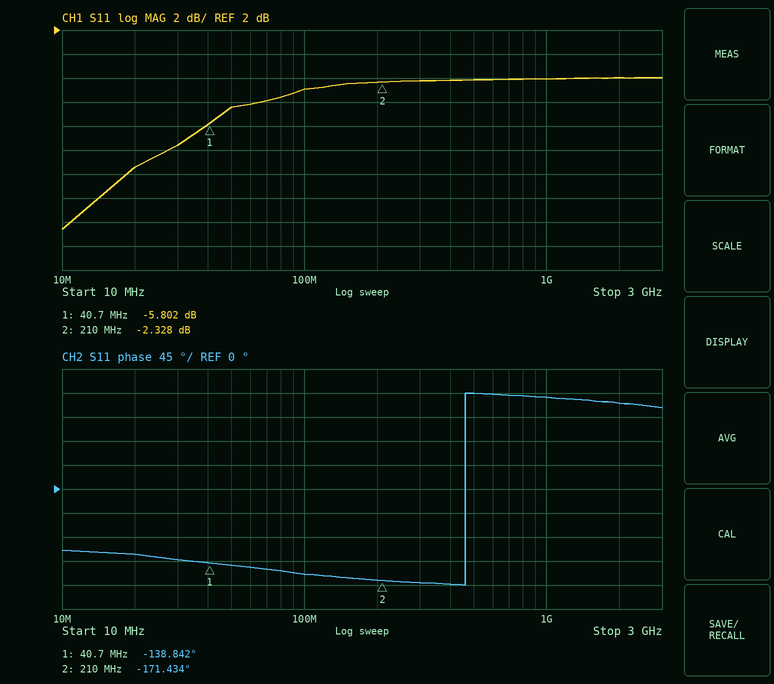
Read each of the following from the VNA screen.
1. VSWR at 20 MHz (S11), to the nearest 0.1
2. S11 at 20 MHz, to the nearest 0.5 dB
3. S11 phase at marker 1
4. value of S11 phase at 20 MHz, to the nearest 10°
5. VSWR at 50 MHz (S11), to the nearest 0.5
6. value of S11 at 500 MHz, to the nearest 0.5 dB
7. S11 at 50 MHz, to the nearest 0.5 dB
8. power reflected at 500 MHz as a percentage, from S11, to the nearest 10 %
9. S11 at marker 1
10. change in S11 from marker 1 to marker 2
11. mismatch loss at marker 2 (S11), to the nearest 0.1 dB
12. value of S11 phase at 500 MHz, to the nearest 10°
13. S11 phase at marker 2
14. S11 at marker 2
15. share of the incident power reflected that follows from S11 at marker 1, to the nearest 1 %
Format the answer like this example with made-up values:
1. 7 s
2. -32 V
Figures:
1. 2.0
2. -9.5 dB
3. -138.842°
4. -120°
5. 4.0
6. -2.0 dB
7. -4.5 dB
8. 60 %
9. -5.802 dB
10. 3.474 dB
11. 3.8 dB
12. 180°
13. -171.434°
14. -2.328 dB
15. 26 %
